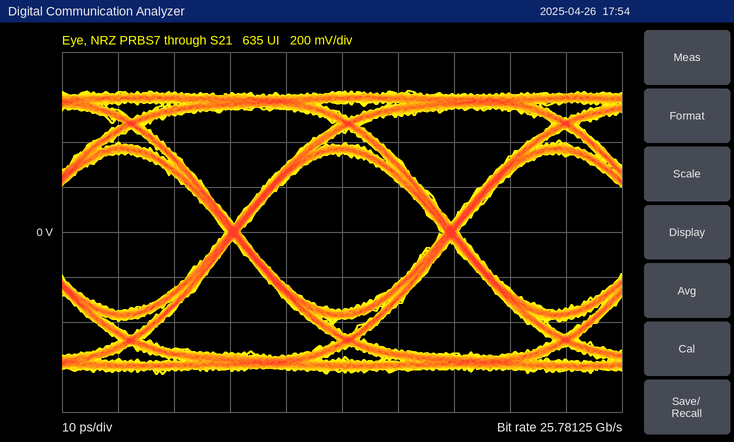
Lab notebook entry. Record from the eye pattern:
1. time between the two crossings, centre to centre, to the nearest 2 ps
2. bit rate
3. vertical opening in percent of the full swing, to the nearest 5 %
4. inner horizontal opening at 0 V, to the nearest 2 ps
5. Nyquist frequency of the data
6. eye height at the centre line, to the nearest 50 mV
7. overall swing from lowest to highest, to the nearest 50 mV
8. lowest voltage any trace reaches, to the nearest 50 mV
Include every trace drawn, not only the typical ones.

38 ps
25.78125 Gb/s
55 %
36 ps
12.89062 GHz
700 mV
1.25 V
-650 mV
